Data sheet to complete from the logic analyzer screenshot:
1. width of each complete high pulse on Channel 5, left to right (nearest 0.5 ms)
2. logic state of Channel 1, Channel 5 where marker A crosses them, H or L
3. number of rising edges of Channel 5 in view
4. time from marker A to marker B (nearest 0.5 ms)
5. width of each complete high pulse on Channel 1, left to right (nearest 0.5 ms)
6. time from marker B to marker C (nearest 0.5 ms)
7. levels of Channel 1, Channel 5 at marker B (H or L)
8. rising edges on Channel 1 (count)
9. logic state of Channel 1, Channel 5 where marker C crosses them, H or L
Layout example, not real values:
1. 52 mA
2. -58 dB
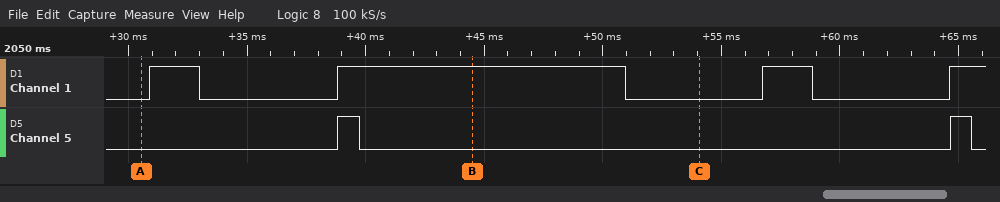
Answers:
1. 1 ms, 1 ms
2. Channel 1=L, Channel 5=L
3. 2
4. 14 ms
5. 2 ms, 12 ms, 2 ms
6. 9.5 ms
7. Channel 1=H, Channel 5=L
8. 4
9. Channel 1=L, Channel 5=L
